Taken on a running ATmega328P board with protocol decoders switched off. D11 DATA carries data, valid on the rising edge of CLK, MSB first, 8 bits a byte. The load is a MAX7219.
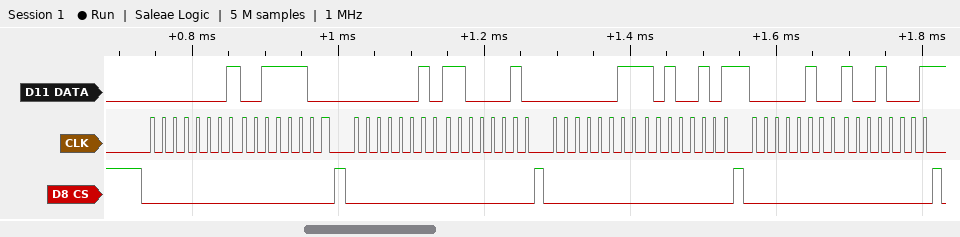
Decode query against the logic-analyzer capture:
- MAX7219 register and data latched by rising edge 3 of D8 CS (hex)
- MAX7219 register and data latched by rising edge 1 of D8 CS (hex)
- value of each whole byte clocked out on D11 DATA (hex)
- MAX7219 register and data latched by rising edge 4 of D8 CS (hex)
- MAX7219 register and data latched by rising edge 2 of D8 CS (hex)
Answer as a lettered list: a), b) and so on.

a) register 0x3, data 0xA5
b) register 0x1, data 0x3C
c) 01 3C 02 C2 03 A5 04 91
d) register 0x4, data 0x91
e) register 0x2, data 0xC2
